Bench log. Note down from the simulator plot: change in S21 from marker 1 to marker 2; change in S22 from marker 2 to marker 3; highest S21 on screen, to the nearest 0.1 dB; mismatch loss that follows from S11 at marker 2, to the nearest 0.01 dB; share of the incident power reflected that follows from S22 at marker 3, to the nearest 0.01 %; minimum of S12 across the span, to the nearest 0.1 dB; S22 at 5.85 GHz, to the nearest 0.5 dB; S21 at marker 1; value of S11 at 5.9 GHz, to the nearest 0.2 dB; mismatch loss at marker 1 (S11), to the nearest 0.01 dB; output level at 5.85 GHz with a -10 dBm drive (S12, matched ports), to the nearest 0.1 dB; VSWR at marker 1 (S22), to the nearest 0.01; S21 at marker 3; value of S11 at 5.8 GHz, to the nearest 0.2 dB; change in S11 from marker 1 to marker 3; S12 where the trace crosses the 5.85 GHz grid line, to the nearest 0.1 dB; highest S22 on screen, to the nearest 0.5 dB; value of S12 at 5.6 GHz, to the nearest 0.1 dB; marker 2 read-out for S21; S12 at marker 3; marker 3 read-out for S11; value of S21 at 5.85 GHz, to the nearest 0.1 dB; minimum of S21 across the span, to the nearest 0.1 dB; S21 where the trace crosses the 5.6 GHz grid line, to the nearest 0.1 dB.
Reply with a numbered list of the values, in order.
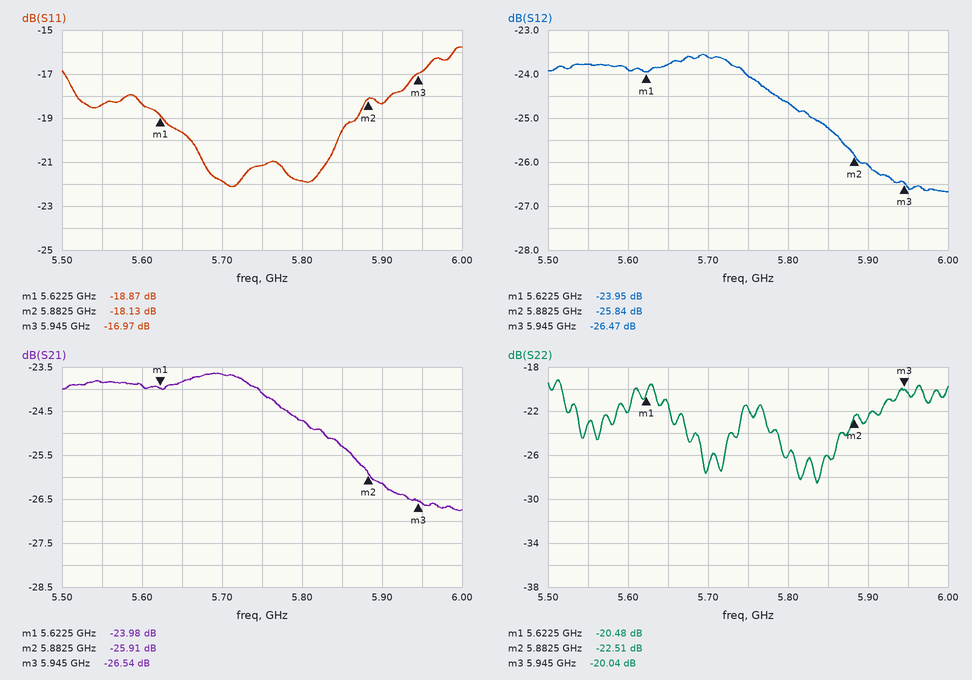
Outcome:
1. -1.93 dB
2. 2.47 dB
3. -23.6 dB
4. 0.07 dB
5. 0.99 %
6. -26.7 dB
7. -26.0 dB
8. -23.98 dB
9. -18.4 dB
10. 0.06 dB
11. -35.2 dBm
12. 1.21
13. -26.54 dB
14. -21.8 dB
15. 1.90 dB
16. -25.2 dB
17. -19.0 dB
18. -23.9 dB
19. -25.91 dB
20. -26.47 dB
21. -16.97 dB
22. -25.3 dB
23. -26.8 dB
24. -23.9 dB
